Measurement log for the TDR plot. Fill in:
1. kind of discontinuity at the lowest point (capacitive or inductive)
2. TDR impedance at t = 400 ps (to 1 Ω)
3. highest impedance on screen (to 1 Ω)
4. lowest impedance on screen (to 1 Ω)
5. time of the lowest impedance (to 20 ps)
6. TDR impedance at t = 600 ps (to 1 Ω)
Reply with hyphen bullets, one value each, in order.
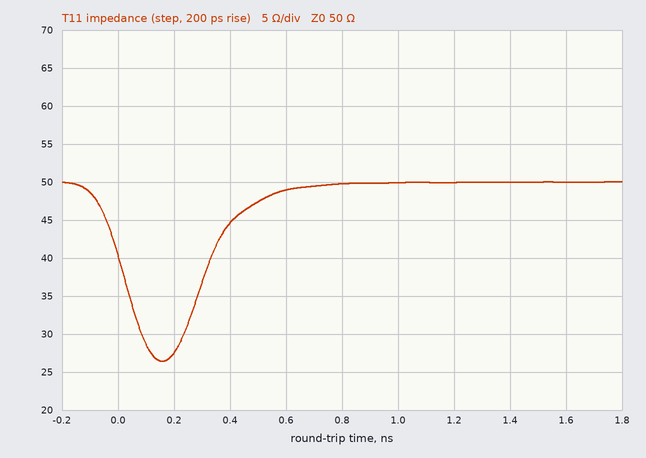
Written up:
- capacitive
- 45 Ω
- 50 Ω
- 26 Ω
- 160 ps
- 49 Ω
